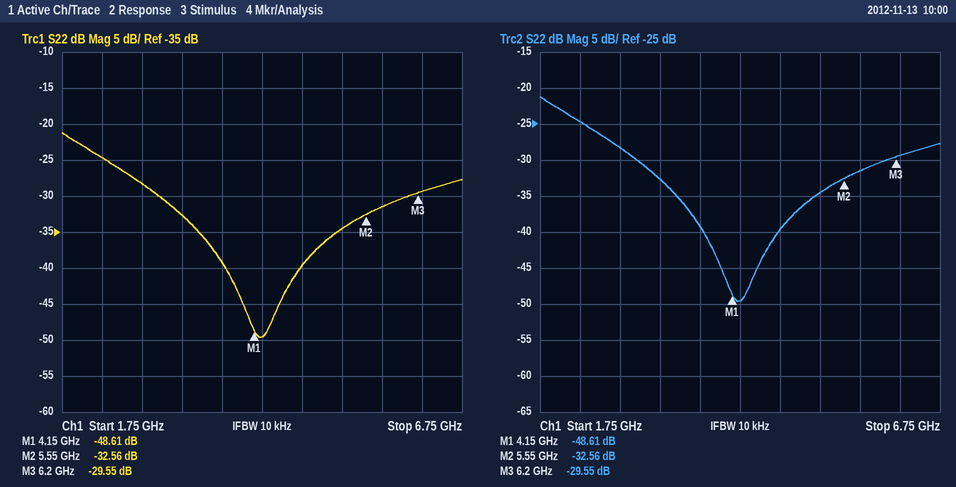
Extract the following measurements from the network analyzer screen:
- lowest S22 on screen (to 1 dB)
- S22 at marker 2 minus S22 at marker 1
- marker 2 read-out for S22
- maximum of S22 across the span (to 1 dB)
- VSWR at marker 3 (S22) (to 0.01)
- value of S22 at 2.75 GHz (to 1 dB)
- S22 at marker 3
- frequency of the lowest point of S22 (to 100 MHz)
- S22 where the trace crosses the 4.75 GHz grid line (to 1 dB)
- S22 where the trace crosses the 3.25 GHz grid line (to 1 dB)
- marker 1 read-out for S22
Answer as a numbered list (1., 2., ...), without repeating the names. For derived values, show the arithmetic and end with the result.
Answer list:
1. -50 dB
2. -32.56 − (-48.61) = 16.05 dB
3. -32.56 dB
4. -21 dB
5. (1 + 0.0333)/(1 − 0.0333) ≈ 1.07
6. -28 dB
7. -29.55 dB
8. 4.2 GHz
9. -40 dB
10. -33 dB
11. -48.61 dB
